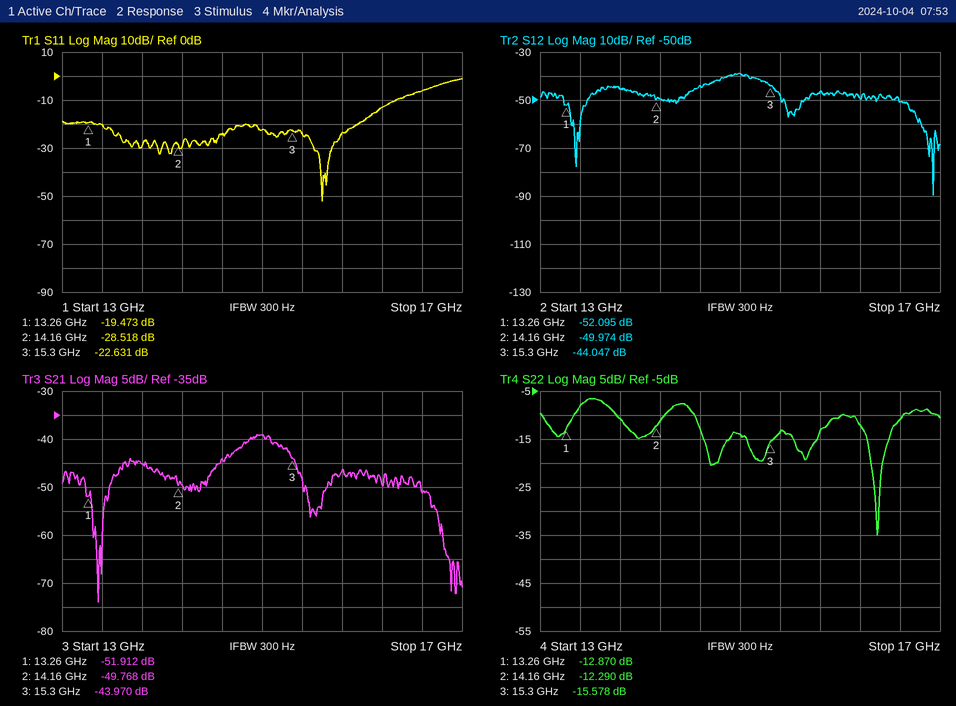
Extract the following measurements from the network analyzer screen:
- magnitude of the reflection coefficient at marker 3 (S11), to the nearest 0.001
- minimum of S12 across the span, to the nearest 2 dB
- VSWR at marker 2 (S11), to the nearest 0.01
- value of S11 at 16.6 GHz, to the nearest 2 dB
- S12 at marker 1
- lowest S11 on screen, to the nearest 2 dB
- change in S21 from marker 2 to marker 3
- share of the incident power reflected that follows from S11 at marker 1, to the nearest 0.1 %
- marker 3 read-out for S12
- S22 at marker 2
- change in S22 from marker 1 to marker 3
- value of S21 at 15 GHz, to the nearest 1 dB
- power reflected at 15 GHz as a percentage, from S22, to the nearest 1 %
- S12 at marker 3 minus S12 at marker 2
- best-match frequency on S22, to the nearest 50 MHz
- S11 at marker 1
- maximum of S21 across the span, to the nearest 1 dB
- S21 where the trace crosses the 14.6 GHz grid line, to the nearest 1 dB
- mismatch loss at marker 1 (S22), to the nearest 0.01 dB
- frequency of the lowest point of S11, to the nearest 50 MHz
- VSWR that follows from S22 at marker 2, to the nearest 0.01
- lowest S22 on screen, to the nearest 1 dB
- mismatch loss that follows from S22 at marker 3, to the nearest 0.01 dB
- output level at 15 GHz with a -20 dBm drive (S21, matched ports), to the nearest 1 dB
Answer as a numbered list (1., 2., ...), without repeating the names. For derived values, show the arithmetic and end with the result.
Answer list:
1. 10^(-22.631/20) ≈ 0.074
2. -90 dB
3. (1 + 0.0375)/(1 − 0.0375) ≈ 1.08
4. -6 dB
5. -52.095 dB
6. -52 dB
7. -43.97 − (-49.768) = 5.798 dB
8. 10^(-19.473/10) ≈ 1.1 %
9. -44.047 dB
10. -12.290 dB
11. -15.578 − (-12.87) = -2.708 dB
12. -39 dB
13. 10^(-14/10) ≈ 4 %
14. -44.047 − (-49.974) = 5.927 dB
15. 16.35 GHz
16. -19.473 dB
17. -39 dB
18. -44 dB
19. −10 log10(1 − 10^(-12.87/10)) ≈ 0.23 dB
20. 15.60 GHz
21. (1 + 0.2429)/(1 − 0.2429) ≈ 1.64
22. -35 dB
23. −10 log10(1 − 10^(-15.578/10)) ≈ 0.12 dB
24. -20 dBm + (-39 dB) = -59 dBm
